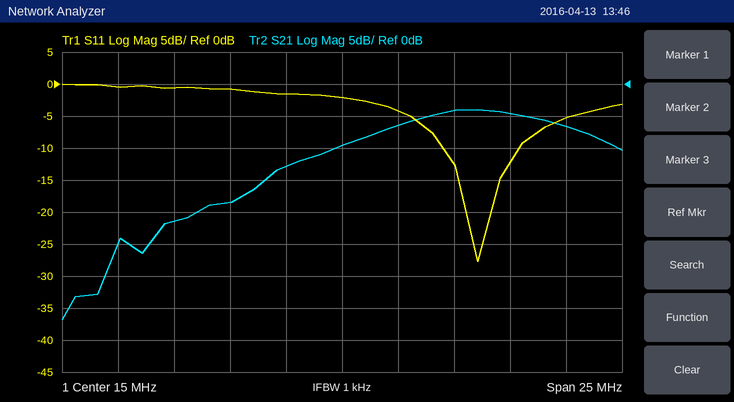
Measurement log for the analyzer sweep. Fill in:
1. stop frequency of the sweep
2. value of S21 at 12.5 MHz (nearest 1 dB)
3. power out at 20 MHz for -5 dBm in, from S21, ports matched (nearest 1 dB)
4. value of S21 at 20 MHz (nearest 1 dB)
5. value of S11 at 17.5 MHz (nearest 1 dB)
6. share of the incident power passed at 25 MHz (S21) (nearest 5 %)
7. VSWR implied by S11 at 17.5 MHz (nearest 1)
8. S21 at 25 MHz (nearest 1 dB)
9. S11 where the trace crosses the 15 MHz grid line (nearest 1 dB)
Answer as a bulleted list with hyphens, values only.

- 27.5 MHz
- -13 dB
- -9 dBm
- -4 dB
- -4 dB
- 20 %
- 4
- -7 dB
- -2 dB
